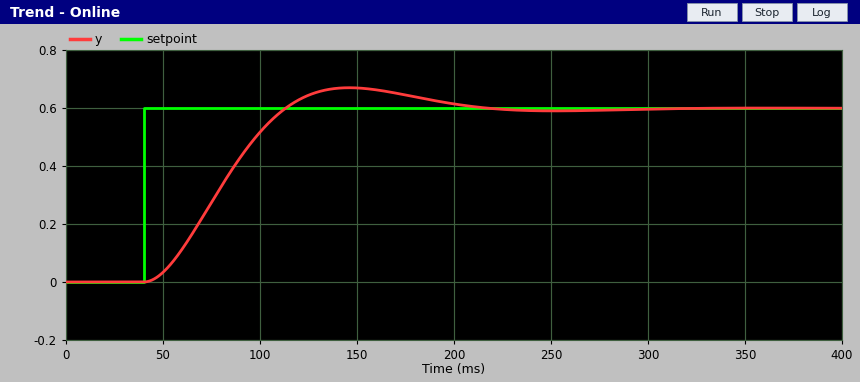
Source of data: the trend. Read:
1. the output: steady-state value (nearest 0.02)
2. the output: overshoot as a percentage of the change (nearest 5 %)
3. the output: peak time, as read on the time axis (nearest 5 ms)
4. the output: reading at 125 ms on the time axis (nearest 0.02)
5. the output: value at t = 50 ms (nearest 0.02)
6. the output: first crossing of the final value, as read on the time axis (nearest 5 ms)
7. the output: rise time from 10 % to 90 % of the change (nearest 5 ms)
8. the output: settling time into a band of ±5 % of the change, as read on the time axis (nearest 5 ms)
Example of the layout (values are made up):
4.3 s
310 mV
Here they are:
0.60
10 %
145 ms
0.64
0.04
115 ms
50 ms
185 ms
